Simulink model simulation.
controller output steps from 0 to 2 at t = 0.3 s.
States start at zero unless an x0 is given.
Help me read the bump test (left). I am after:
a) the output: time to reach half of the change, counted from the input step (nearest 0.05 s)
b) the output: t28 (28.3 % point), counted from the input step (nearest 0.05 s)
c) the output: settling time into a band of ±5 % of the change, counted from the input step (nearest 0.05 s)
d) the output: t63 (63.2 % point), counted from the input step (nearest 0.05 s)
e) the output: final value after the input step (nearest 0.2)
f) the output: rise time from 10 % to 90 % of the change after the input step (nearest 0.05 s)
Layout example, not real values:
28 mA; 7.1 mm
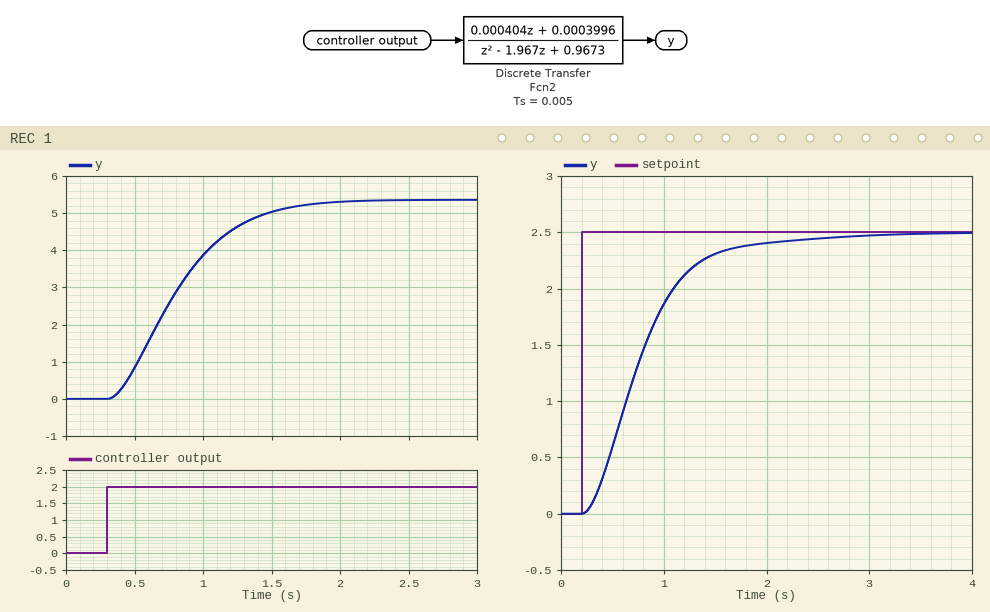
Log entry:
0.45 s; 0.30 s; 1.25 s; 0.60 s; 5.4; 0.90 s
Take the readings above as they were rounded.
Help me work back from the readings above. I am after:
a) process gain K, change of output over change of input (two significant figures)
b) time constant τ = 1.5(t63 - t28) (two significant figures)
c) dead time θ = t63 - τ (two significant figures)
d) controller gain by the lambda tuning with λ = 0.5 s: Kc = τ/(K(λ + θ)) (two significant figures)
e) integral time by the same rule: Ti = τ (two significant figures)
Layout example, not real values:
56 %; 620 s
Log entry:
2.7; 0.45 s; 0.15 s; 0.26; 0.45 s
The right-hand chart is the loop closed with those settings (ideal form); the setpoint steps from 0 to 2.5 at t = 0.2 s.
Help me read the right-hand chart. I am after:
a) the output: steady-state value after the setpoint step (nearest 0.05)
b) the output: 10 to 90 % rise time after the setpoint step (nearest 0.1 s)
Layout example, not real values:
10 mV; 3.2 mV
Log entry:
2.50; 1.0 s
